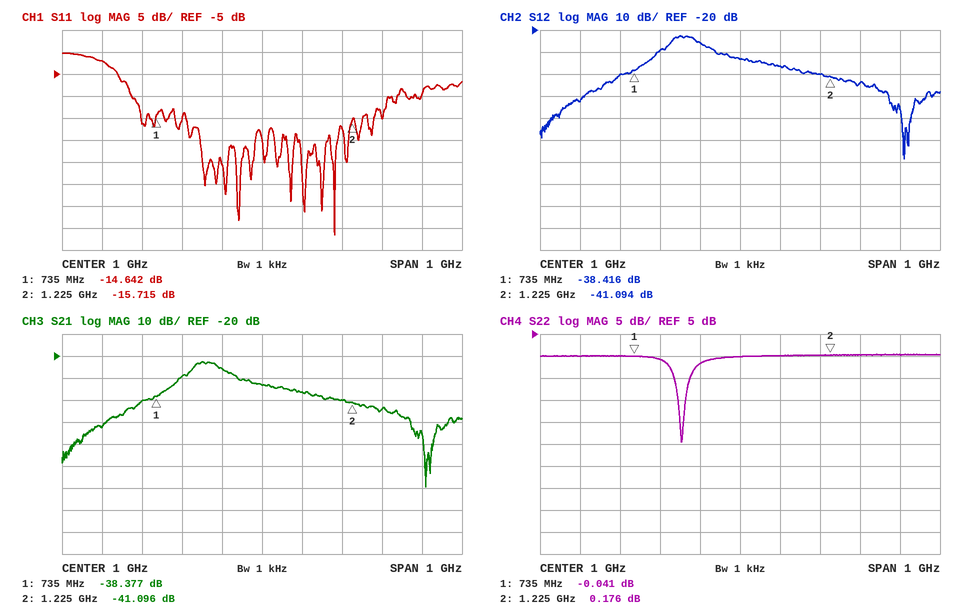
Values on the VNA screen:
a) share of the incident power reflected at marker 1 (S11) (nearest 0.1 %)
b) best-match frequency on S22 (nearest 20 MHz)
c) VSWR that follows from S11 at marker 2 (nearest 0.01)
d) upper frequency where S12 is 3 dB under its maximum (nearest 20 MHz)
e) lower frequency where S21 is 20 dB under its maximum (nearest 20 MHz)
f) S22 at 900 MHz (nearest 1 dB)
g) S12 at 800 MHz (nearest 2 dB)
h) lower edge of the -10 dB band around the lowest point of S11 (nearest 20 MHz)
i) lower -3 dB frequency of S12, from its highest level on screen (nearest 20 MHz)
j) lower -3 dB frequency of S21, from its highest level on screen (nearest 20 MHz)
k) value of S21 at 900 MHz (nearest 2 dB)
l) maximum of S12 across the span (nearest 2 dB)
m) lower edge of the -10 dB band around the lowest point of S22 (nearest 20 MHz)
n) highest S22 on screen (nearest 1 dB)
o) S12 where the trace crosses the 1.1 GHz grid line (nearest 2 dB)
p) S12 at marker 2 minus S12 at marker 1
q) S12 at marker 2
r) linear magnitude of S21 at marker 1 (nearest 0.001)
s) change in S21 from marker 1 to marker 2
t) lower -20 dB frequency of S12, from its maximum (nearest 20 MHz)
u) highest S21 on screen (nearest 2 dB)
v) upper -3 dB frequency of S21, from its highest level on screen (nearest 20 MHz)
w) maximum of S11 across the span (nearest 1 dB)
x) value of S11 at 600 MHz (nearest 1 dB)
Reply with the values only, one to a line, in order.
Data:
3.4 %
860 MHz
1.39
900 MHz
680 MHz
-2 dB
-30 dB
680 MHz
820 MHz
820 MHz
-26 dB
-22 dB
840 MHz
0 dB
-36 dB
-2.678 dB
-41.094 dB
0.012
-2.719 dB
680 MHz
-22 dB
900 MHz
0 dB
-2 dB
